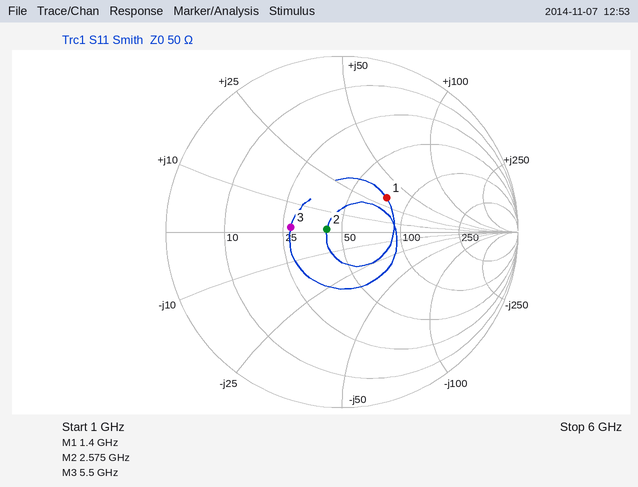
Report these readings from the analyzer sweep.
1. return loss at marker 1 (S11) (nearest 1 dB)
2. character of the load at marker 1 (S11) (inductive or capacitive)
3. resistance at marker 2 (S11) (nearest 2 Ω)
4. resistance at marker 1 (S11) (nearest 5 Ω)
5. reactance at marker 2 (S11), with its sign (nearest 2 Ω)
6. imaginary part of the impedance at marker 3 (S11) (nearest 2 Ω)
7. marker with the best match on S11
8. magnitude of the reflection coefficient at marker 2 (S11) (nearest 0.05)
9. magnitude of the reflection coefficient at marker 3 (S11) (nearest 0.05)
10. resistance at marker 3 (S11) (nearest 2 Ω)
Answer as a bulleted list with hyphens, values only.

- 10 dB
- inductive
- 42 Ω
- 75 Ω
- +2 Ω
- +2 Ω
- marker 2
- 0.10
- 0.30
- 28 Ω
